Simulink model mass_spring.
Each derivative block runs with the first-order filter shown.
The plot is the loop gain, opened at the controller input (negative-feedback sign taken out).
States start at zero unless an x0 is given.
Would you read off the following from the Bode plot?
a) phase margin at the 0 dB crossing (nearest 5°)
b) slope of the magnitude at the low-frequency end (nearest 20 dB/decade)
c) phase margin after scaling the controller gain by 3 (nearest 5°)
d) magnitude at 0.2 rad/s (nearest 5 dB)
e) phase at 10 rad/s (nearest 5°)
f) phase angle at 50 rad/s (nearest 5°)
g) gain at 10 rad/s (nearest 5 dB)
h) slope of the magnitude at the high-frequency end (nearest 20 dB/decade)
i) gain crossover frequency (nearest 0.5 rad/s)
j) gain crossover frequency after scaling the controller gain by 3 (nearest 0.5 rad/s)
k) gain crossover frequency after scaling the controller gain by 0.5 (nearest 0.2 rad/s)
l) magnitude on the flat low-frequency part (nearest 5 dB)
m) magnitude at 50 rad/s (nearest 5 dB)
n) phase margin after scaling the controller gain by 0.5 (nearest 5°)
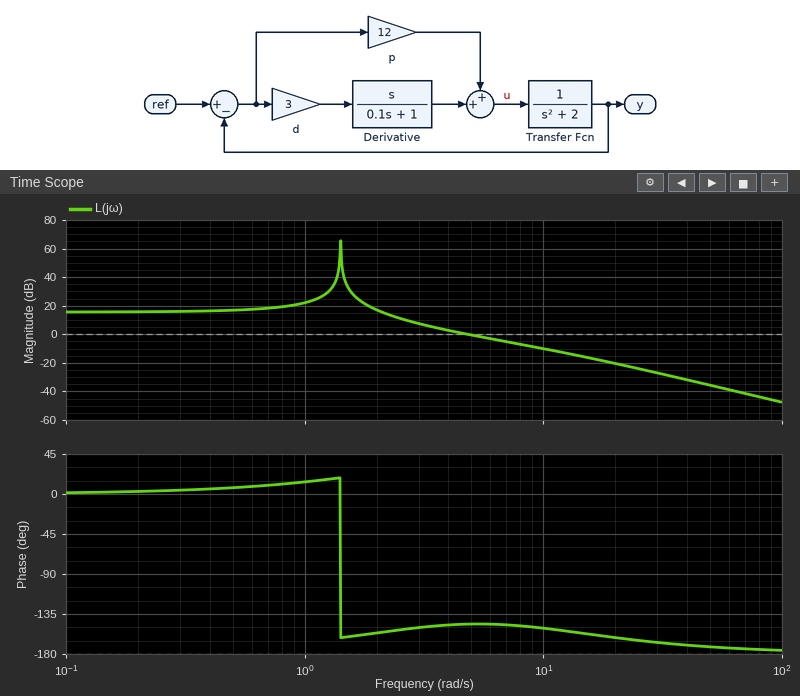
35°
0 dB/decade
30°
15 dB
-150°
-170°
-10 dB
-40 dB/decade
5.0 rad/s
9.5 rad/s
3.2 rad/s
15 dB
-35 dB
30°
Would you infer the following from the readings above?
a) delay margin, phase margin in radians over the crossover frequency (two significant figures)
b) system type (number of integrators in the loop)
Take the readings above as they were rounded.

0.12 s
0
